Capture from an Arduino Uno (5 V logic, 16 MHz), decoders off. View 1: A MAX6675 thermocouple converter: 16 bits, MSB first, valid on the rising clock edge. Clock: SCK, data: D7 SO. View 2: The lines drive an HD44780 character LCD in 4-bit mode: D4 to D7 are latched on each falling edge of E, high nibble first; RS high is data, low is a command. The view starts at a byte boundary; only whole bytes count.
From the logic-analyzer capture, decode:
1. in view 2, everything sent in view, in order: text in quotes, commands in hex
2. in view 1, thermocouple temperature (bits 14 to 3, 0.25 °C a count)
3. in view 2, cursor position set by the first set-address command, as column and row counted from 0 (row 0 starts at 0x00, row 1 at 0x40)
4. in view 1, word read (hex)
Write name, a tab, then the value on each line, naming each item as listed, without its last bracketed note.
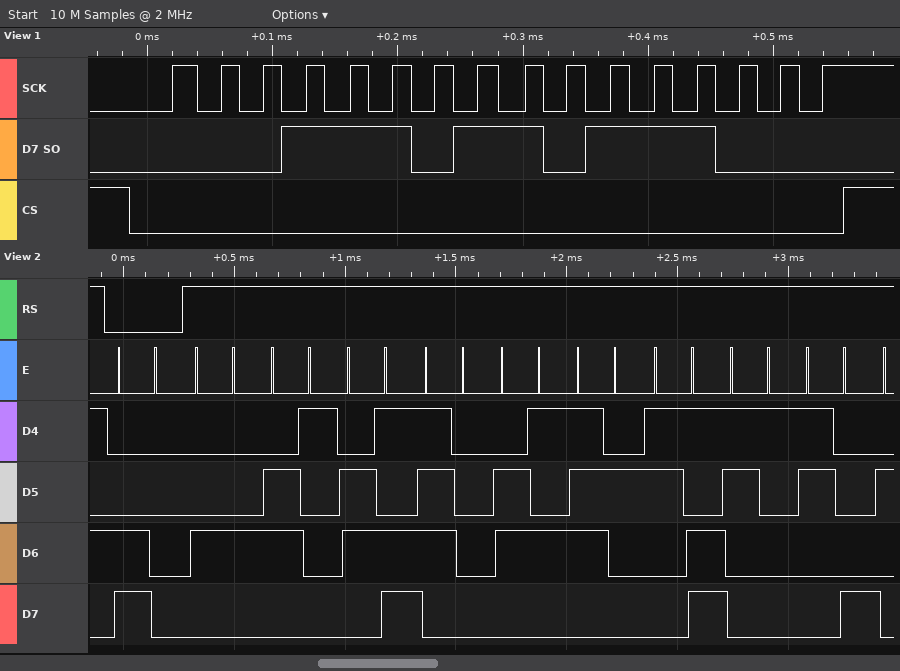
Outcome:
in view 2, everything sent in view, in order: text in quotes, commands in hex	0xC0 "Damper=18"
in view 1, thermocouple temperature	237.75 °C
in view 2, cursor position set by the first set-address command, as column and row counted from 0	column 0, row 1
in view 1, word read	0x1DB8
